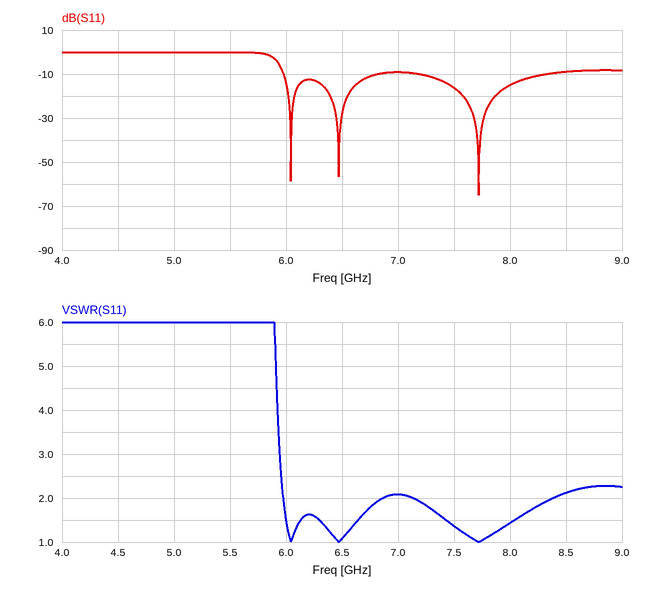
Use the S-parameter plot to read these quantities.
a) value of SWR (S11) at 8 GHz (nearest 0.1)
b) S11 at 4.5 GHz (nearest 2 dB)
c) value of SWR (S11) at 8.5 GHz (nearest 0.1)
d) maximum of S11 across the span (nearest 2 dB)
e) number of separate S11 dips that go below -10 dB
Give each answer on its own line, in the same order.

1.4
0 dB
2.1
0 dB
3
